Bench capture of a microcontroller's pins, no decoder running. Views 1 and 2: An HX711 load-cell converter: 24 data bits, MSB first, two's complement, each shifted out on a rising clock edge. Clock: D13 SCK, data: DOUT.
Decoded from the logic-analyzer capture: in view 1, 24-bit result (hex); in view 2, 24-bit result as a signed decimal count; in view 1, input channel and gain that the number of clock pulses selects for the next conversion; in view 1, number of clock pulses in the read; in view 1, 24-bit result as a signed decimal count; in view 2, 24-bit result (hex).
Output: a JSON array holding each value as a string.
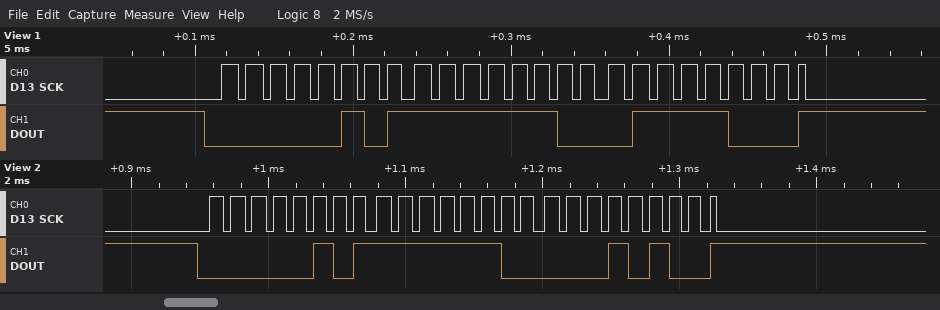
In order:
["0x05FC78", "392212", "channel A, gain 128", "25", "392312", "0x05FC14"]
